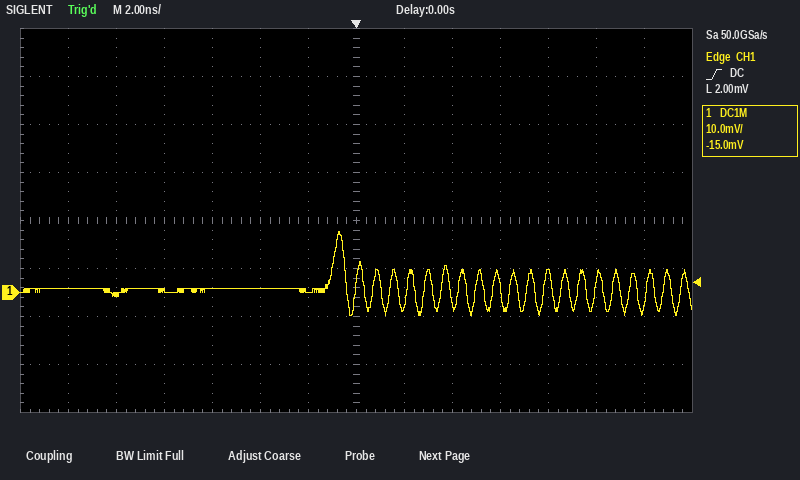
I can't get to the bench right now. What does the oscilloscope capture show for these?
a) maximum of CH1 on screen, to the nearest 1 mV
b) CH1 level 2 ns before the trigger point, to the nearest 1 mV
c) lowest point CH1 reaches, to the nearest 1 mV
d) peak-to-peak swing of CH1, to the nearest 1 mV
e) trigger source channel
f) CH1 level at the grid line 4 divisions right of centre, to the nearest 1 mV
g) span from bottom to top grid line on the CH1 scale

13 mV
0 mV
-5 mV
18 mV
CH1
4 mV
80 mV
